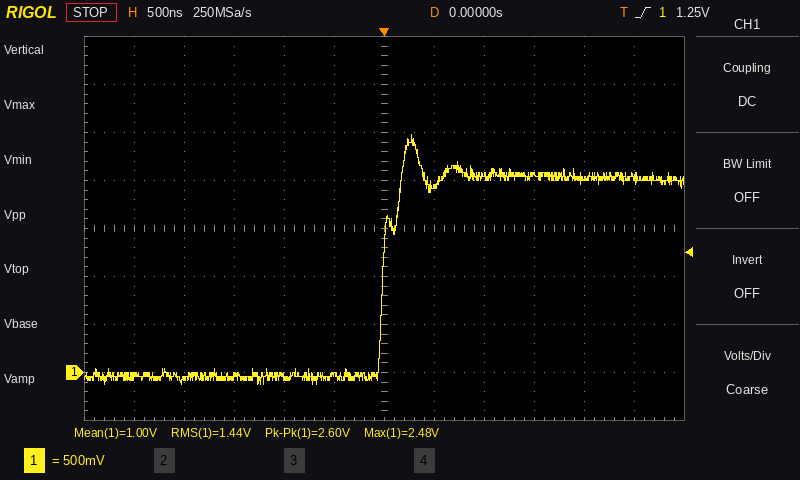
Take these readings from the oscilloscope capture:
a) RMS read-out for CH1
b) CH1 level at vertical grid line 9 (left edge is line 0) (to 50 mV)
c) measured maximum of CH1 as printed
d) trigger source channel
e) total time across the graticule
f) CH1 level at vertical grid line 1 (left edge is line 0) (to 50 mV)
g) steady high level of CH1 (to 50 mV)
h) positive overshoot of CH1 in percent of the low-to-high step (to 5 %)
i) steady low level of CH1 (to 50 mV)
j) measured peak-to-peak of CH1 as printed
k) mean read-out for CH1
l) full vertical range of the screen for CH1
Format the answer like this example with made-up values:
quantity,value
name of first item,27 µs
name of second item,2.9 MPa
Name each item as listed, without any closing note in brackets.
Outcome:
quantity,value
RMS read-out for CH1,1.44 V
CH1 level at vertical grid line 9 (left edge is line 0),2.05 V
measured maximum of CH1 as printed,2.48 V
trigger source channel,CH1
total time across the graticule,6 µs
CH1 level at vertical grid line 1 (left edge is line 0),-50 mV
steady high level of CH1,2.05 V
positive overshoot of CH1 in percent of the low-to-high step,20 %
steady low level of CH1,-50 mV
measured peak-to-peak of CH1 as printed,2.60 V
mean read-out for CH1,1.00 V
full vertical range of the screen for CH1,4 V
